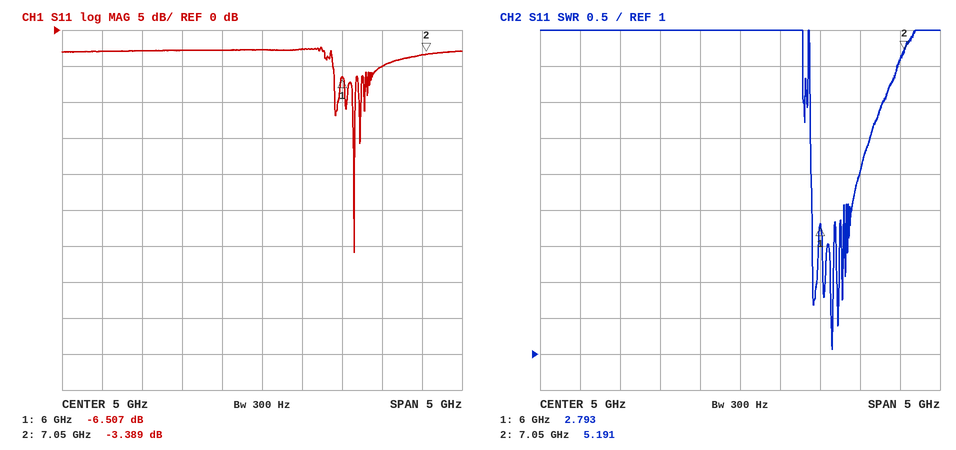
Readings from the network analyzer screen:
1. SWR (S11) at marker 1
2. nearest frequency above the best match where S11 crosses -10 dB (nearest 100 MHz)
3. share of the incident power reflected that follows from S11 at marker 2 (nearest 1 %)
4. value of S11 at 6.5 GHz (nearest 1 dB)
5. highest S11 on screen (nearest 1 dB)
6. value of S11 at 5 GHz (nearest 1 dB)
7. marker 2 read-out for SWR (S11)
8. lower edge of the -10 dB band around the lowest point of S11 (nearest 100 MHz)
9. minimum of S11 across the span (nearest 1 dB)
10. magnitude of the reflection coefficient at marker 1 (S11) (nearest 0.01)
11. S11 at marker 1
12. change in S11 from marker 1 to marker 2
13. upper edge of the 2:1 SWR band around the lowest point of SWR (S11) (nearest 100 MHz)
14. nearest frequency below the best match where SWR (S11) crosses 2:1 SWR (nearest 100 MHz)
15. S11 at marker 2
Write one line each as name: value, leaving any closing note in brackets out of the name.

SWR (S11) at marker 1: 2.793
nearest frequency above the best match where S11 crosses -10 dB: 6.2 GHz
share of the incident power reflected that follows from S11 at marker 2: 46 %
value of S11 at 6.5 GHz: -5 dB
highest S11 on screen: -2 dB
value of S11 at 5 GHz: -3 dB
marker 2 read-out for SWR: 5.191
lower edge of the -10 dB band around the lowest point of S11: 6.1 GHz
minimum of S11 across the span: -31 dB
magnitude of the reflection coefficient at marker 1 (S11): 0.47
S11 at marker 1: -6.507 dB
change in S11 from marker 1 to marker 2: 3.118 dB
upper edge of the 2:1 SWR band around the lowest point of SWR (S11): 6.2 GHz
nearest frequency below the best match where SWR (S11) crosses 2:1 SWR: 6.1 GHz
S11 at marker 2: -3.389 dB
